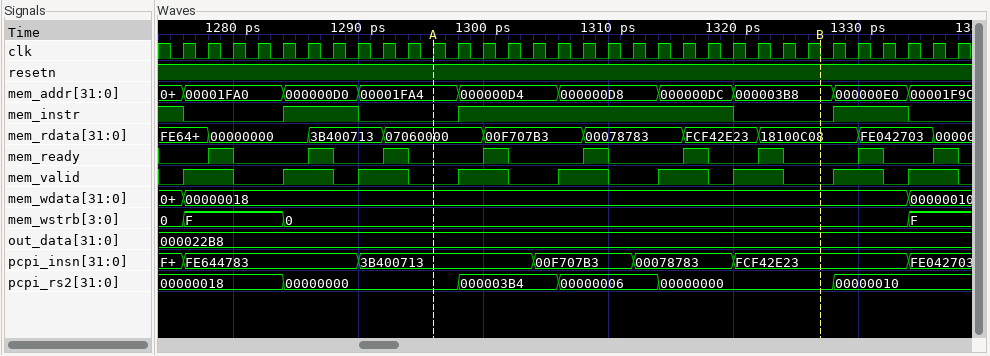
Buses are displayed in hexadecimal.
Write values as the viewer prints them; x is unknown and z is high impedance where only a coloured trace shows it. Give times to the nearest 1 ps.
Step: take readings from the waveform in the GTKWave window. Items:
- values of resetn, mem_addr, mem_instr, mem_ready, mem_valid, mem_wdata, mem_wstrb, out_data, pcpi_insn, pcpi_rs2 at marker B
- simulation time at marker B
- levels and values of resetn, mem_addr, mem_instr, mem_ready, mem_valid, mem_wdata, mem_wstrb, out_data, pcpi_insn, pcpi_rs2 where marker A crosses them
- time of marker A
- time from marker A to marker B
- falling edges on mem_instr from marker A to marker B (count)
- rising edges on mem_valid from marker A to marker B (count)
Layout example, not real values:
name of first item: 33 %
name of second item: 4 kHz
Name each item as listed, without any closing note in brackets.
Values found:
values of resetn, mem_addr, mem_instr, mem_ready, mem_valid, mem_wdata, mem_wstrb, out_data, pcpi_insn, pcpi_rs2 at marker B: resetn=1, mem_addr=000003B8, mem_instr=0, mem_ready=0, mem_valid=0, mem_wdata=00000018, mem_wstrb=0, out_data=000022B8, pcpi_insn=FCF42E23, pcpi_rs2=00000000
simulation time at marker B: 1327 ps
levels and values of resetn, mem_addr, mem_instr, mem_ready, mem_valid, mem_wdata, mem_wstrb, out_data, pcpi_insn, pcpi_rs2 where marker A crosses them: resetn=1, mem_addr=00001FA4, mem_instr=0, mem_ready=0, mem_valid=0, mem_wdata=00000018, mem_wstrb=0, out_data=000022B8, pcpi_insn=3B400713, pcpi_rs2=00000000
time of marker A: 1296 ps
time from marker A to marker B: 31 ps
falling edges on mem_instr from marker A to marker B: 1
rising edges on mem_valid from marker A to marker B: 4
